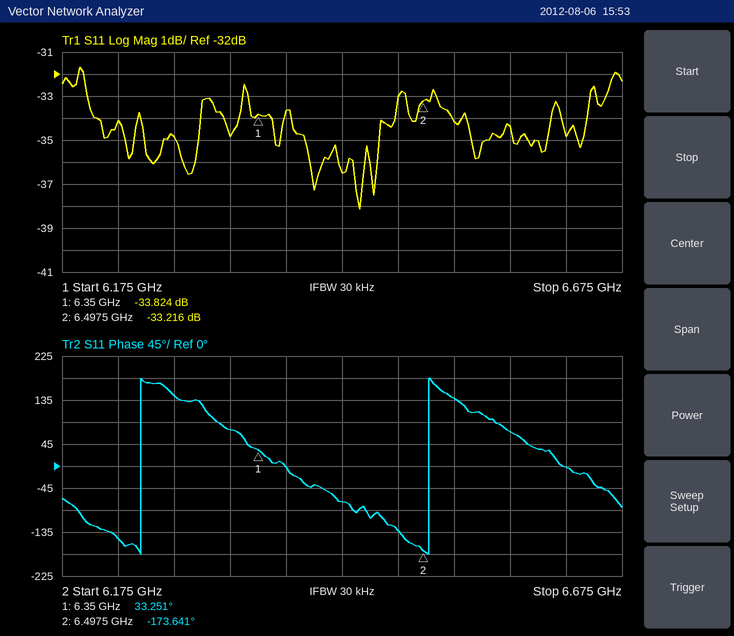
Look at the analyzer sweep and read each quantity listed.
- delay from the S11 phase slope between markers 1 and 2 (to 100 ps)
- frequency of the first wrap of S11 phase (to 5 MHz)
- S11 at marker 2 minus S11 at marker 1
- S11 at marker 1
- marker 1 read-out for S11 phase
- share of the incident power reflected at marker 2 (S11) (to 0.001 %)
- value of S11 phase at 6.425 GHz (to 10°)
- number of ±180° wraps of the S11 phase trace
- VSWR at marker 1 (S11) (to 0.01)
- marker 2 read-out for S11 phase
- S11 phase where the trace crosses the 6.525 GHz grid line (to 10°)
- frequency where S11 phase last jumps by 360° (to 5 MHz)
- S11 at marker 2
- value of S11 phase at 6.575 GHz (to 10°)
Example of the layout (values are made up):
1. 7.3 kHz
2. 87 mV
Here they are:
1. 3.9 ns
2. 6.245 GHz
3. 0.608 dB
4. -33.824 dB
5. 33.251°
6. 0.048 %
7. -70°
8. 2
9. 1.04
10. -173.641°
11. 140°
12. 6.500 GHz
13. -33.216 dB
14. 70°
